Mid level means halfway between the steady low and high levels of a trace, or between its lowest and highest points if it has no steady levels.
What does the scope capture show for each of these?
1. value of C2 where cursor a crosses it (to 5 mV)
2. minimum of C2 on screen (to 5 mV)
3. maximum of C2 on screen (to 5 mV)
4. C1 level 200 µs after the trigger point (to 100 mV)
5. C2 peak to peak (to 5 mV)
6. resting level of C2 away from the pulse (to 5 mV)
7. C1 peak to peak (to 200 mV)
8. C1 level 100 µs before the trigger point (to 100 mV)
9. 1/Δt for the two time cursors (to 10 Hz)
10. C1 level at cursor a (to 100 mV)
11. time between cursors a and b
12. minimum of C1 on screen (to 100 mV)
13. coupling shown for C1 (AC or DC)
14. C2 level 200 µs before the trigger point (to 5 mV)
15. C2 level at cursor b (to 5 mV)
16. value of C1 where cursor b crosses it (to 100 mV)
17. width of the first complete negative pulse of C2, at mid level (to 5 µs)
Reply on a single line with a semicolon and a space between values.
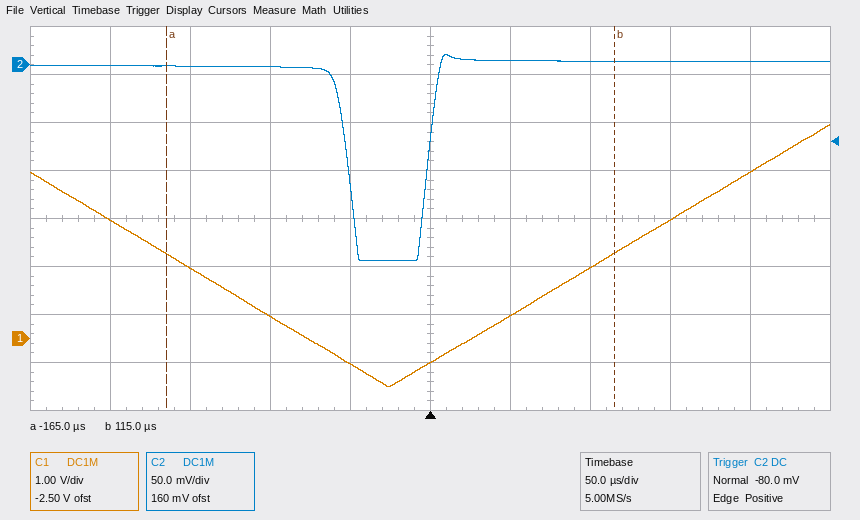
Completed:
0 mV; -205 mV; 10 mV; 3.5 V; 215 mV; 5 mV; 5.4 V; 500 mV; 3.57 kHz; 1.8 V; 280 µs; -1.0 V; DC; 0 mV; 5 mV; 1.8 V; 50 µs
